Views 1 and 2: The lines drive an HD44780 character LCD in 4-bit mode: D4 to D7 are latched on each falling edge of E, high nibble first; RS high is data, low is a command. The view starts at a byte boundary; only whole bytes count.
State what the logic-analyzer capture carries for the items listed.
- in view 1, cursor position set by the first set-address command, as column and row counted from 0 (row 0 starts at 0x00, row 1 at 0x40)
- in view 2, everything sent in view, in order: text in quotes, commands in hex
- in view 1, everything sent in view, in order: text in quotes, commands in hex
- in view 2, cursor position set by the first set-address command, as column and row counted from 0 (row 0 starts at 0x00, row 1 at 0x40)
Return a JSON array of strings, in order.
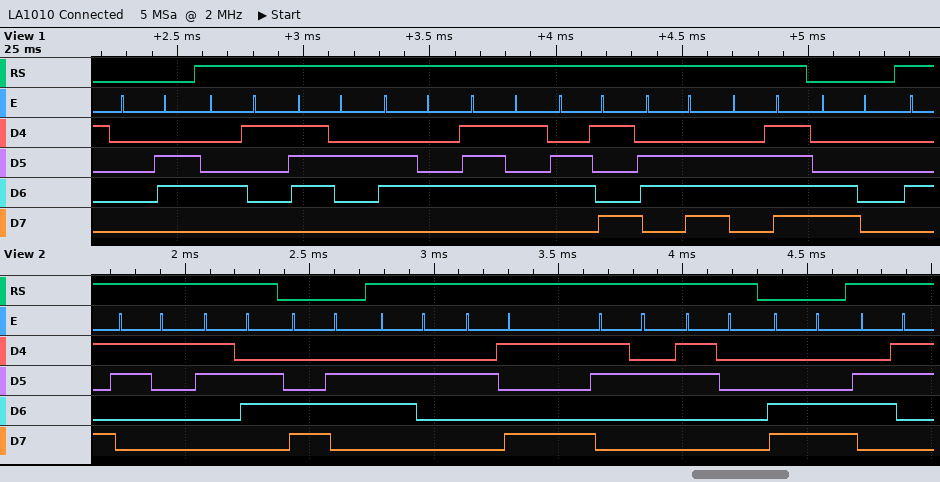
["column 0, row 1", "\"16\" 0xC6 \"b)20\" 0xCC \"c\"", "0x06 \"Arduino\" 0xC0", "column 6, row 1"]
